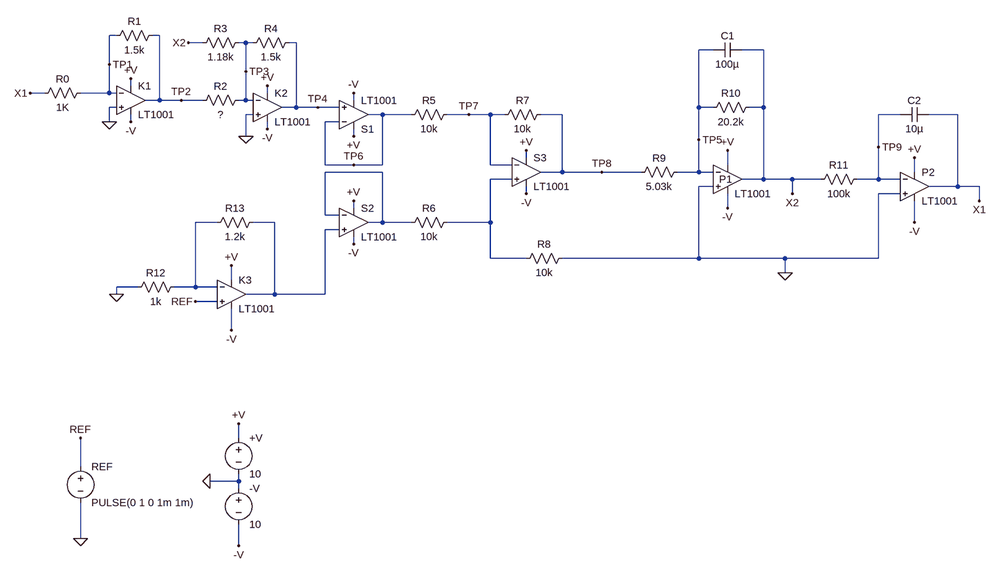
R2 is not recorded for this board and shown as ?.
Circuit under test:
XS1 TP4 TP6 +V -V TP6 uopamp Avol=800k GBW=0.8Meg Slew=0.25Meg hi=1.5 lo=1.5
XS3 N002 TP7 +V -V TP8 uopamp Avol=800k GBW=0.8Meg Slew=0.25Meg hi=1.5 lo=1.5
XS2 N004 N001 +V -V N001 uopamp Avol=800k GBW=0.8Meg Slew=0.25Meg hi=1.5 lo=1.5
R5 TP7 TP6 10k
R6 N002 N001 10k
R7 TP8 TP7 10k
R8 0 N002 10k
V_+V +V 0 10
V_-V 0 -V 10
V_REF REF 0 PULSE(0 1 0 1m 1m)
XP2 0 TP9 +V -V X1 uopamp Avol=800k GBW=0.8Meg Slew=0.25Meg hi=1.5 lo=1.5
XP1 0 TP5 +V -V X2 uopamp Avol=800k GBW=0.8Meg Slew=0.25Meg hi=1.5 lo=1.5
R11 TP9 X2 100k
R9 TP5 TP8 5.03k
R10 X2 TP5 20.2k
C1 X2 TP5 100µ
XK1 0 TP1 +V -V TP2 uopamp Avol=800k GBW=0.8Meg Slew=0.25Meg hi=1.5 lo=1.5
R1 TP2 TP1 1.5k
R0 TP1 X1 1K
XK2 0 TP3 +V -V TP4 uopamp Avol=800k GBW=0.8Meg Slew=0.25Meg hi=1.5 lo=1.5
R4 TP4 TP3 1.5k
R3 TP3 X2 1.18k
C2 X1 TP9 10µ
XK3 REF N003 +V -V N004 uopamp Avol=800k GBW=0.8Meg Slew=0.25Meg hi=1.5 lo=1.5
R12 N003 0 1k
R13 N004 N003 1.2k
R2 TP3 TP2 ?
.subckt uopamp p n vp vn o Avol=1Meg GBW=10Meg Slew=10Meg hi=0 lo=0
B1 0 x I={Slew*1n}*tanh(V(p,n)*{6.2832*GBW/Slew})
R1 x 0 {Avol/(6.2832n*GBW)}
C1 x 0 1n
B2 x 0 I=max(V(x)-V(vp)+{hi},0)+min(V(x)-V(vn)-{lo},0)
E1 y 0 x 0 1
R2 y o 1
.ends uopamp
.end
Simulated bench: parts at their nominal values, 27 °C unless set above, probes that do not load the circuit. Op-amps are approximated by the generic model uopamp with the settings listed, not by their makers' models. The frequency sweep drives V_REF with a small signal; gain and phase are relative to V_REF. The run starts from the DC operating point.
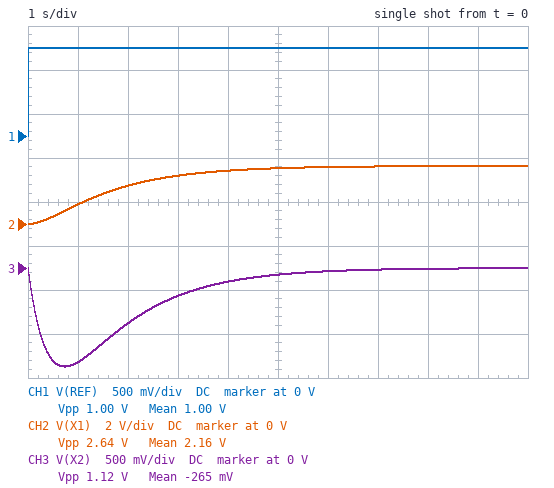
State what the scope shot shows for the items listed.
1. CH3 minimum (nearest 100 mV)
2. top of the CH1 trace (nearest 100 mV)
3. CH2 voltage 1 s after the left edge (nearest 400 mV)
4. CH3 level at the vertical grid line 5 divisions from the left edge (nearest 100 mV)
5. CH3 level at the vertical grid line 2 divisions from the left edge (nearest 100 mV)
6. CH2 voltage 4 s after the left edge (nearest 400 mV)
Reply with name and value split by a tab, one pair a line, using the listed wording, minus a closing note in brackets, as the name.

CH3 minimum	-1.1 V
top of the CH1 trace	1.0 V
CH2 voltage 1 s after the left edge	800 mV
CH3 level at the vertical grid line 5 divisions from the left edge	-100 mV
CH3 level at the vertical grid line 2 divisions from the left edge	-600 mV
CH2 voltage 4 s after the left edge	2.4 V
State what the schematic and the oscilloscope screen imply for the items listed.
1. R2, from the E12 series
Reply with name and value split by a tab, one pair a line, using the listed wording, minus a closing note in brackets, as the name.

R2, from the E12 series	2.7 kΩ
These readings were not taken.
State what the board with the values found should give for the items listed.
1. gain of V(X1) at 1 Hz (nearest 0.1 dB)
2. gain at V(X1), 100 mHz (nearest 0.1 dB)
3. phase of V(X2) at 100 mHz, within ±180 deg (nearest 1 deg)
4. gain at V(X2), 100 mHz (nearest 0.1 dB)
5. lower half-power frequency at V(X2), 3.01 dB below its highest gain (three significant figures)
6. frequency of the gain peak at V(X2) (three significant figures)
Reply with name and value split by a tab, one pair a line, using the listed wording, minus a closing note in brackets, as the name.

gain of V(X1) at 1 Hz	-19.7 dB
gain at V(X1), 100 mHz	5.7 dB
phase of V(X2) at 100 mHz, within ±180 deg	-146 deg
gain at V(X2), 100 mHz	1.6 dB
lower half-power frequency at V(X2), 3.01 dB below its highest gain	75.4 mHz
frequency of the gain peak at V(X2)	205 mHz
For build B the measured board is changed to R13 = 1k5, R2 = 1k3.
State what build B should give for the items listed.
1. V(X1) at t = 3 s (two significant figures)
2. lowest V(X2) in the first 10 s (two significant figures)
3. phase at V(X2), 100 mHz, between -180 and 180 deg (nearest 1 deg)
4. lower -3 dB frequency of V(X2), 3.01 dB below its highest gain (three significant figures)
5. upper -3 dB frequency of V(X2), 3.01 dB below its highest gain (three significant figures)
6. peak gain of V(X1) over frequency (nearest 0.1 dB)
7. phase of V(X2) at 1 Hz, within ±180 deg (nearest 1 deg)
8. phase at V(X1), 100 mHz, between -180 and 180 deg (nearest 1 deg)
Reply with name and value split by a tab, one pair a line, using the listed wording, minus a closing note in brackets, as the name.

V(X1) at t = 3 s	1.5 V
lowest V(X2) in the first 10 s	-1.1 V
phase at V(X2), 100 mHz, between -180 and 180 deg	-122 deg
lower -3 dB frequency of V(X2), 3.01 dB below its highest gain	140 mHz
upper -3 dB frequency of V(X2), 3.01 dB below its highest gain	621 mHz
peak gain of V(X1) over frequency	3.2 dB
phase of V(X2) at 1 Hz, within ±180 deg	118 deg
phase at V(X1), 100 mHz, between -180 and 180 deg	-32 deg
